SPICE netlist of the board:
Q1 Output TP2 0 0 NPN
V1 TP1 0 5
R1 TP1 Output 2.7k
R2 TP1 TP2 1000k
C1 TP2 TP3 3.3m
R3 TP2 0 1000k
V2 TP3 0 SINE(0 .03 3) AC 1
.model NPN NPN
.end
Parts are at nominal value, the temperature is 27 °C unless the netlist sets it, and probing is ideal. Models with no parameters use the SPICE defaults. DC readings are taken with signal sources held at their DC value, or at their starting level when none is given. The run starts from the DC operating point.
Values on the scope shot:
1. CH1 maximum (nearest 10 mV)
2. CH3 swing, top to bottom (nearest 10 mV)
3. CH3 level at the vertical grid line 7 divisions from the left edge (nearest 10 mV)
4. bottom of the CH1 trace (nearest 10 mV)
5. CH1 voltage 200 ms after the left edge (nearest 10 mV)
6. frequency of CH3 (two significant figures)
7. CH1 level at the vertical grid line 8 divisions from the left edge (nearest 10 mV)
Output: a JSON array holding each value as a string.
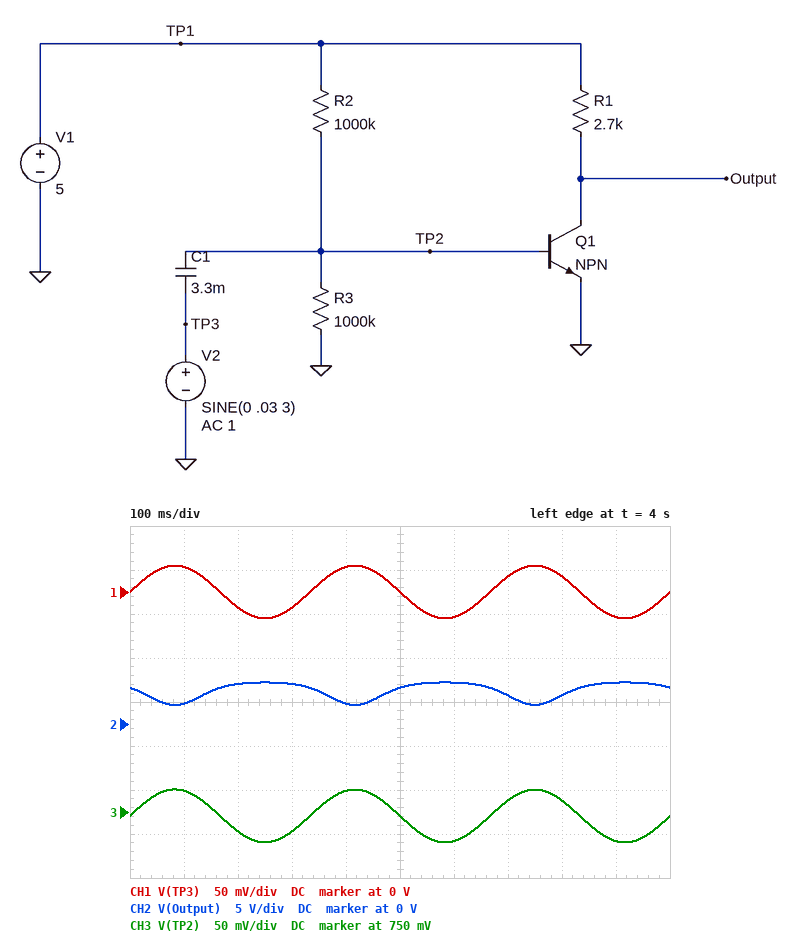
["30 mV", "60 mV", "760 mV", "-30 mV", "-20 mV", "3.0 Hz", "20 mV"]
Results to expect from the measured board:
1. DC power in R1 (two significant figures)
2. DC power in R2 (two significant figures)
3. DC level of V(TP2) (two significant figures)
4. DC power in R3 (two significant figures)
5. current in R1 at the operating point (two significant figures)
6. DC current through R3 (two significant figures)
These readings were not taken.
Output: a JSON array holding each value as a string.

["330 µW", "18 µW", "750 mV", "560 nW", "350 µA", "750 nA"]
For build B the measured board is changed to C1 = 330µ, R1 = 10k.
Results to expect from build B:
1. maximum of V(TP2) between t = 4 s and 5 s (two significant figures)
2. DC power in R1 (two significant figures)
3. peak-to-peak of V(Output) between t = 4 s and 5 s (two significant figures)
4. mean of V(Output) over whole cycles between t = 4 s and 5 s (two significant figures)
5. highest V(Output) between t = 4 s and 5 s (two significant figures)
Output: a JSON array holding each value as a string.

["760 mV", "1.2 mW", "4.4 V", "2.8 V", "4.5 V"]
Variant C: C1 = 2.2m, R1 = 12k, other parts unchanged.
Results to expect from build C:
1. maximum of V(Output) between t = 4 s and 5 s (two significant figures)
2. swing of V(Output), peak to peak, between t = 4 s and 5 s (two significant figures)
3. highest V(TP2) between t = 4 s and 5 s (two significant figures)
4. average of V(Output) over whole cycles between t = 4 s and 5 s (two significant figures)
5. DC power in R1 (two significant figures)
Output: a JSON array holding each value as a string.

["4.5 V", "4.4 V", "750 mV", "2.7 V", "1.5 mW"]
